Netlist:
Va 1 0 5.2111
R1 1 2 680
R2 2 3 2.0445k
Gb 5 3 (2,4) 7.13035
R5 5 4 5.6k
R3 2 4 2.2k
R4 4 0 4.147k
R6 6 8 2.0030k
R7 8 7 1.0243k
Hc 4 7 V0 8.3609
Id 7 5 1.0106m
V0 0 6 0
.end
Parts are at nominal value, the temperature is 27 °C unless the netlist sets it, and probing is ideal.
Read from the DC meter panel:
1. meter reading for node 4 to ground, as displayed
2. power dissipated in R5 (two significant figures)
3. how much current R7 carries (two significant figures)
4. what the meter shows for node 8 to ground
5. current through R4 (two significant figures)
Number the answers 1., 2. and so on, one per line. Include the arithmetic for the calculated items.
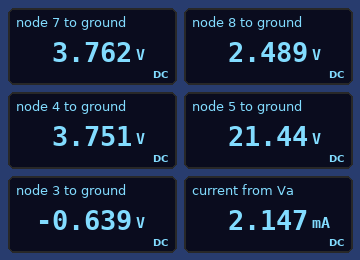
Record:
1. 3.751 V
2. (21.44 V - 3.751 V)^2 / 5.6 kΩ = 56 mW
3. (3.762 V - 2.489 V) / 1.024 kΩ = 1.2 mA
4. 2.489 V
5. (3.751 V) / 4.147 kΩ = 900 µA
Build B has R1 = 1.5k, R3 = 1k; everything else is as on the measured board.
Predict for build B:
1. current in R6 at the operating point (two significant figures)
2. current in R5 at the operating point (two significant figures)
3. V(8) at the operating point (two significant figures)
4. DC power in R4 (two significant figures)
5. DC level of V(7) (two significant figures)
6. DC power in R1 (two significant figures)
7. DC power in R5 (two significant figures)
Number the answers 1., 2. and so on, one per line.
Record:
1. 930 µA
2. 2.6 mA
3. 1.9 V
4. 1.9 mW
5. 2.8 V
6. 3.9 mW
7. 38 mW
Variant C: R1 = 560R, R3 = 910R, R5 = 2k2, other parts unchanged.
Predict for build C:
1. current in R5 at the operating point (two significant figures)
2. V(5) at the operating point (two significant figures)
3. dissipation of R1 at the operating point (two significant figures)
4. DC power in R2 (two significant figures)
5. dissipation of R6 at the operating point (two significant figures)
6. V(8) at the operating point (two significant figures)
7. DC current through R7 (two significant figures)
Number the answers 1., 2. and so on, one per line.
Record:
1. 3.3 mA
2. 11 V
3. 2.9 mW
4. 10 mW
5. 3.4 mW
6. 2.6 V
7. 1.3 mA
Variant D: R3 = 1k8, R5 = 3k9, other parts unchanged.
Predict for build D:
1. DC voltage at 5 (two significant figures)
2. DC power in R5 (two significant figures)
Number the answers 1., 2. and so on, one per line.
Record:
1. 16 V
2. 39 mW
